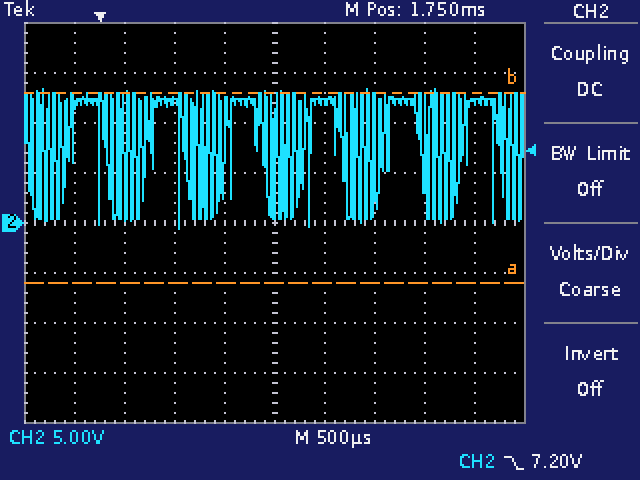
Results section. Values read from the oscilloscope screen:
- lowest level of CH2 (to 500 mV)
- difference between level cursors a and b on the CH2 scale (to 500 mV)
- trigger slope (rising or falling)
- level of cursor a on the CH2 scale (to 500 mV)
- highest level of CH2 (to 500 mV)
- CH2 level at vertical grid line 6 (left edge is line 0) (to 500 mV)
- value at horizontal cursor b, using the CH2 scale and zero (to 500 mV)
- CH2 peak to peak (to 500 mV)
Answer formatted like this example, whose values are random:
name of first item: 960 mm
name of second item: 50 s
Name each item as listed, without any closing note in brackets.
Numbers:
lowest level of CH2: -500 mV
difference between level cursors a and b on the CH2 scale: 19.0 V
trigger slope: falling
level of cursor a on the CH2 scale: -6.0 V
highest level of CH2: 13.5 V
CH2 level at vertical grid line 6 (left edge is line 0): 12.0 V
value at horizontal cursor b, using the CH2 scale and zero: 13.0 V
CH2 peak to peak: 14.0 V
